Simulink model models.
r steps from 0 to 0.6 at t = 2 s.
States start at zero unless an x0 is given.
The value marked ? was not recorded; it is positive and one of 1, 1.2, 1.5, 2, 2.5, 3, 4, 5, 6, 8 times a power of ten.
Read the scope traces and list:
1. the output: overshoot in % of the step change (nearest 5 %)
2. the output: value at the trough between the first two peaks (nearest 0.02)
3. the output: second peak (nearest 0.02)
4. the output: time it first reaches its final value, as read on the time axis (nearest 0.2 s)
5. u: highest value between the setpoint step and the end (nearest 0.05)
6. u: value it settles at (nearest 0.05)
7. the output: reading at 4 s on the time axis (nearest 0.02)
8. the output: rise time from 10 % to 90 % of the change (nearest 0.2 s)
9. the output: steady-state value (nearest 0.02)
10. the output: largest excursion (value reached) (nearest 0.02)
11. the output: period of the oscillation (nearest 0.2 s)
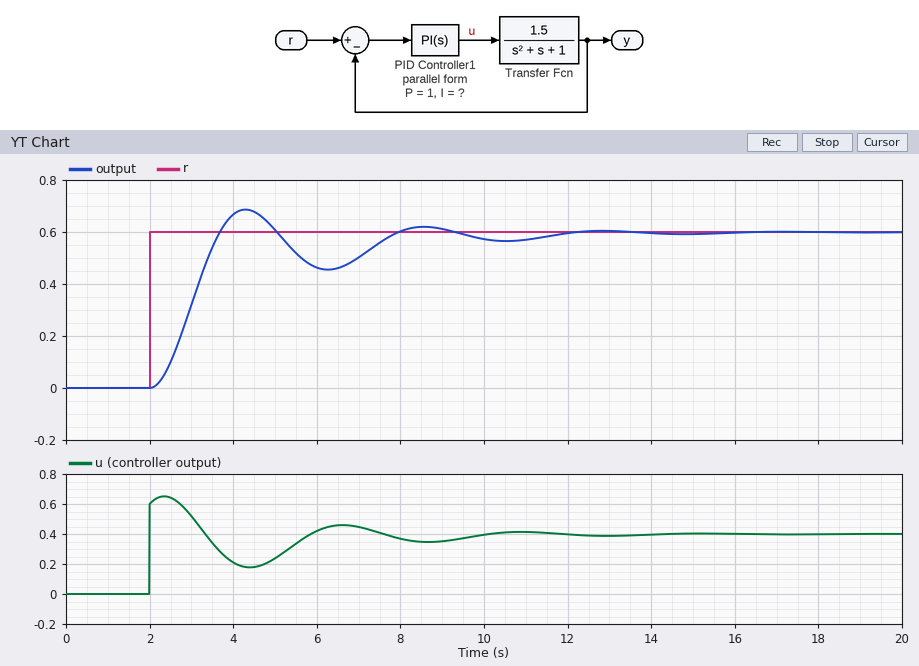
15 %
0.46
0.62
3.6 s
0.65
0.40
0.66
1.2 s
0.60
0.68
4.2 s
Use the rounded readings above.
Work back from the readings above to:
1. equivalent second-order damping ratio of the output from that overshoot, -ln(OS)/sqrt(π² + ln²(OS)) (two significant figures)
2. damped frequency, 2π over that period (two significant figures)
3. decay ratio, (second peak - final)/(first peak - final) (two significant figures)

0.52
1.5 rad/s
0.25
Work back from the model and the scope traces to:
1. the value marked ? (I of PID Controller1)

0.5
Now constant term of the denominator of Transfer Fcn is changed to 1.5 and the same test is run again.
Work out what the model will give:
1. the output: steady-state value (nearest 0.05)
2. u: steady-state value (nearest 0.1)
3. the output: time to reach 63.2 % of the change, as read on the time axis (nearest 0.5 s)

0.60
0.6
3.0 s
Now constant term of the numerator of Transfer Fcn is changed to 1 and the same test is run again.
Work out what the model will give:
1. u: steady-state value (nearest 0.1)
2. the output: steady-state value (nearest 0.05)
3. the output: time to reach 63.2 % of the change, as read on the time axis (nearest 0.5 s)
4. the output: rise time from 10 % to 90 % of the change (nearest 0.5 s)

0.6
0.60
3.5 s
1.5 s
